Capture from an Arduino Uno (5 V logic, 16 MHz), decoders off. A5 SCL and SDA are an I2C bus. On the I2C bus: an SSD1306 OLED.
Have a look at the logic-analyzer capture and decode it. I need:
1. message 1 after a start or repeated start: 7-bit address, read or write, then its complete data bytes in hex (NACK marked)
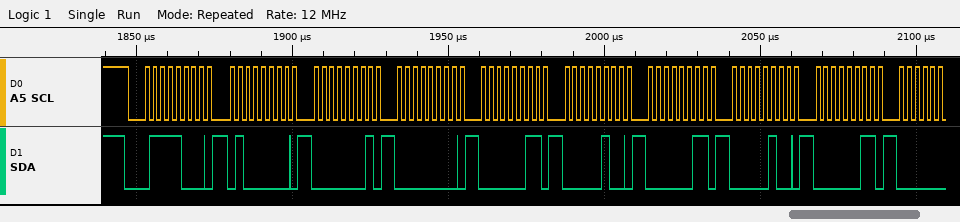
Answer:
0x3C write: 40 01 00 03 04 03 04 03
